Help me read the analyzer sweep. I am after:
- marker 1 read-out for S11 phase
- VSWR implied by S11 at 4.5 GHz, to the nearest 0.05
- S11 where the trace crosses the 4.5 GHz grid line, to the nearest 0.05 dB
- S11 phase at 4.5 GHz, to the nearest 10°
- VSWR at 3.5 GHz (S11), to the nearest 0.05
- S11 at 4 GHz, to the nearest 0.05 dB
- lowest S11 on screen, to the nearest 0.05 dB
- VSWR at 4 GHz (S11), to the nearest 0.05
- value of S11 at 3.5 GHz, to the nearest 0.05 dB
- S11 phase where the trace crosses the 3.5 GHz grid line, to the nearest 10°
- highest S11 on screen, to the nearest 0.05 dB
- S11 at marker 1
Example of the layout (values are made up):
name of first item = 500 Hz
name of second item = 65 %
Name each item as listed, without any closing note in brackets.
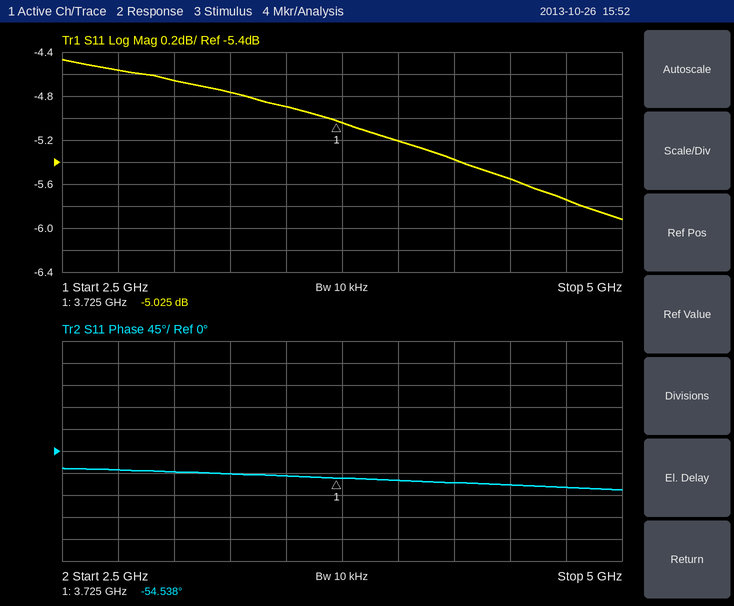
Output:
marker 1 read-out for S11 phase = -54.538°
VSWR implied by S11 at 4.5 GHz, to the nearest 0.05 = 3.25
S11 where the trace crosses the 4.5 GHz grid line, to the nearest 0.05 dB = -5.55 dB
S11 phase at 4.5 GHz, to the nearest 10° = -70°
VSWR at 3.5 GHz (S11), to the nearest 0.05 = 3.65
S11 at 4 GHz, to the nearest 0.05 dB = -5.20 dB
lowest S11 on screen, to the nearest 0.05 dB = -5.90 dB
VSWR at 4 GHz (S11), to the nearest 0.05 = 3.45
value of S11 at 3.5 GHz, to the nearest 0.05 dB = -4.90 dB
S11 phase where the trace crosses the 3.5 GHz grid line, to the nearest 10° = -50°
highest S11 on screen, to the nearest 0.05 dB = -4.45 dB
S11 at marker 1 = -5.025 dB
